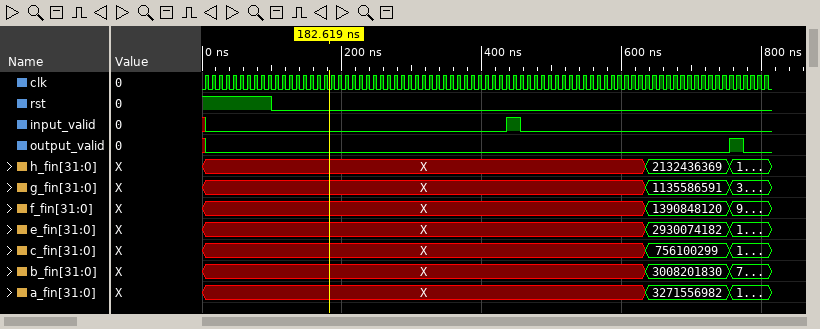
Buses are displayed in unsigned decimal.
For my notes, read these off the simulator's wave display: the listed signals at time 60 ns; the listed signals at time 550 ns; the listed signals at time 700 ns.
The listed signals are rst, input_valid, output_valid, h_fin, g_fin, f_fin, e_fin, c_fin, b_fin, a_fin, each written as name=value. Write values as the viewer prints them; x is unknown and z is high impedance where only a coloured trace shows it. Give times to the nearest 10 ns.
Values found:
rst=1, input_valid=0, output_valid=0, h_fin=X, g_fin=X, f_fin=X, e_fin=X, c_fin=X, b_fin=X, a_fin=X
rst=0, input_valid=0, output_valid=0, h_fin=X, g_fin=X, f_fin=X, e_fin=X, c_fin=X, b_fin=X, a_fin=X
rst=0, input_valid=0, output_valid=0, h_fin=2132436369, g_fin=1135586591, f_fin=1390848120, e_fin=2930074182, c_fin=756100299, b_fin=3008201830, a_fin=3271556982
